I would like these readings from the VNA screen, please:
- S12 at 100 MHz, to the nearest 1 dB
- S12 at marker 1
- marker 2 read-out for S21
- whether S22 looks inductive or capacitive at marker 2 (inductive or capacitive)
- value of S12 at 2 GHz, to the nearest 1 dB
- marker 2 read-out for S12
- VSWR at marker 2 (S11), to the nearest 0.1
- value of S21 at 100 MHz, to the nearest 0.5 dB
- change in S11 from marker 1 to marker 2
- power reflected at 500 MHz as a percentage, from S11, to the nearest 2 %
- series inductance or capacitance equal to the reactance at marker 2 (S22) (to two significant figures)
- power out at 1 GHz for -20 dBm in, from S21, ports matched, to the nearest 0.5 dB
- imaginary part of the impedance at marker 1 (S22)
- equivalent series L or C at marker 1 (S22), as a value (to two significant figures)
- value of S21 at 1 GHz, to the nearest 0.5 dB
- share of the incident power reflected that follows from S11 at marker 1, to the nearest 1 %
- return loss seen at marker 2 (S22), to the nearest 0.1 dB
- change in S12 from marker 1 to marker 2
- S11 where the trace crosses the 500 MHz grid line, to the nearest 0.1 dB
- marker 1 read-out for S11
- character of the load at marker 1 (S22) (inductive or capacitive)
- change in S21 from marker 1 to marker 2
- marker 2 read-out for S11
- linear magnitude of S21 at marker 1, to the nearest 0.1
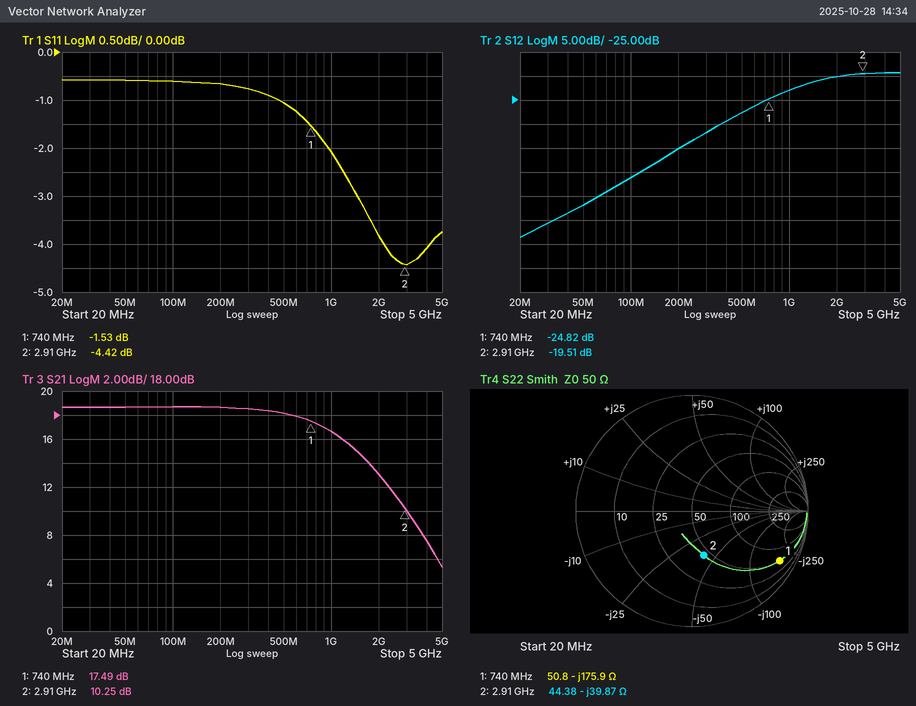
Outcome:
-41 dB
-24.82 dB
10.25 dB
capacitive
-20 dB
-19.51 dB
4.0
18.5 dB
-2.89 dB
78 %
1.4 pF
-3.5 dBm
-175.9 Ω
1.2 pF
16.5 dB
70 %
8.1 dB
5.31 dB
-1.1 dB
-1.53 dB
capacitive
-7.24 dB
-4.42 dB
7.5
